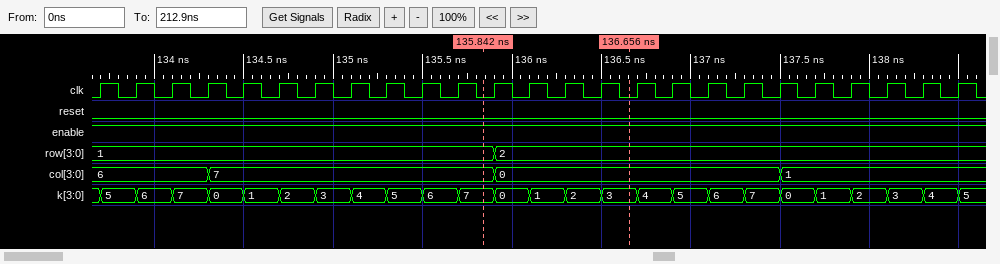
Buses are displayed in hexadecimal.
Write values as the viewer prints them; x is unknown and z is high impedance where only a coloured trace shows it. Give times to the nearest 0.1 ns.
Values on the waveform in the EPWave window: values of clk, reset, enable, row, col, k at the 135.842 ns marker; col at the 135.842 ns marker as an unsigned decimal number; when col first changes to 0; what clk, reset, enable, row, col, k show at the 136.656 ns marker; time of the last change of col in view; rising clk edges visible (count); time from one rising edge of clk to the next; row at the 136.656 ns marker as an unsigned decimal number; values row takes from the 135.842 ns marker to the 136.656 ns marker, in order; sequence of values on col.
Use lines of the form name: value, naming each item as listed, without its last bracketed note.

values of clk, reset, enable, row, col, k at the 135.842 ns marker: clk=0, reset=0, enable=1, row=1, col=7, k=7
col at the 135.842 ns marker as an unsigned decimal number: 7
when col first changes to 0: 135.9 ns
what clk, reset, enable, row, col, k show at the 136.656 ns marker: clk=0, reset=0, enable=1, row=2, col=0, k=3
time of the last change of col in view: 137.5 ns
rising clk edges visible: 25
time from one rising edge of clk to the next: 0.2 ns
row at the 136.656 ns marker as an unsigned decimal number: 2
values row takes from the 135.842 ns marker to the 136.656 ns marker, in order: 1, 2
sequence of values on col: 6, 7, 0, 1
